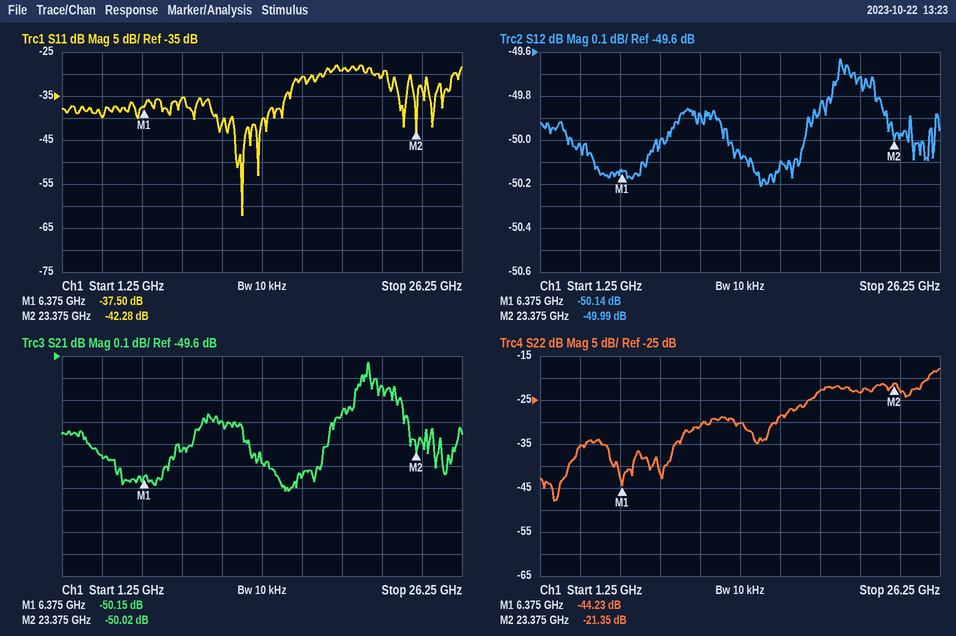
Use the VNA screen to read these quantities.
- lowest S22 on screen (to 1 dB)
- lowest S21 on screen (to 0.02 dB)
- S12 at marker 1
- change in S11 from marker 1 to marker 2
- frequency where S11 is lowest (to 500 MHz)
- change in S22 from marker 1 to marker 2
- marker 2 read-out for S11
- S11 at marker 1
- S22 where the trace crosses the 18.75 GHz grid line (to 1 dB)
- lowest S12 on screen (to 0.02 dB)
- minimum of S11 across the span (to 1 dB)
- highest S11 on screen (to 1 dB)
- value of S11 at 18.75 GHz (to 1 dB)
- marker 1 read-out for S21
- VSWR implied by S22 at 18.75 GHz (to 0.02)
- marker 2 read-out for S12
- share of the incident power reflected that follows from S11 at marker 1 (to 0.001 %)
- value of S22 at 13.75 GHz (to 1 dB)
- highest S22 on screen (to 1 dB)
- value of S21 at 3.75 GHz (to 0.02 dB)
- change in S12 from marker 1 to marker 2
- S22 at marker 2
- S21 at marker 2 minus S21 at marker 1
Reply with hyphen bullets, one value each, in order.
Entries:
- -48 dB
- -50.22 dB
- -50.14 dB
- -4.78 dB
- 12.5 GHz
- 22.88 dB
- -42.28 dB
- -37.50 dB
- -23 dB
- -50.20 dB
- -62 dB
- -28 dB
- -29 dB
- -50.15 dB
- 1.16
- -49.99 dB
- 0.018 %
- -30 dB
- -18 dB
- -50.06 dB
- 0.15 dB
- -21.35 dB
- 0.13 dB
